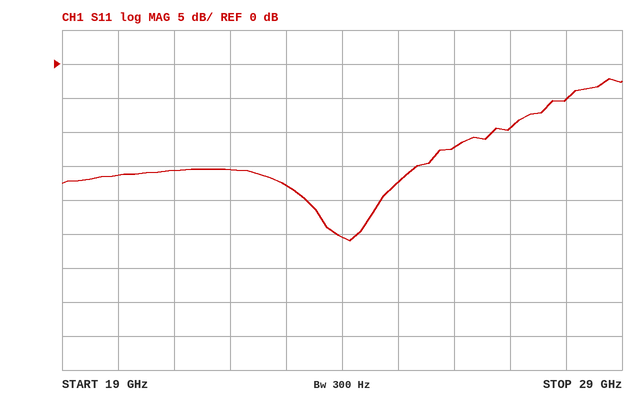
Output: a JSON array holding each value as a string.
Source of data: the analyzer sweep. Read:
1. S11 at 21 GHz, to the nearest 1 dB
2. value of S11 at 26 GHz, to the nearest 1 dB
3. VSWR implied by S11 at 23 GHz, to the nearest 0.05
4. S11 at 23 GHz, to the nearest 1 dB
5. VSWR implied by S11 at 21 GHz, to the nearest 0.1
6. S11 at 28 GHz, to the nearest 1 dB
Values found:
["-16 dB", "-12 dB", "1.30", "-18 dB", "1.4", "-5 dB"]
